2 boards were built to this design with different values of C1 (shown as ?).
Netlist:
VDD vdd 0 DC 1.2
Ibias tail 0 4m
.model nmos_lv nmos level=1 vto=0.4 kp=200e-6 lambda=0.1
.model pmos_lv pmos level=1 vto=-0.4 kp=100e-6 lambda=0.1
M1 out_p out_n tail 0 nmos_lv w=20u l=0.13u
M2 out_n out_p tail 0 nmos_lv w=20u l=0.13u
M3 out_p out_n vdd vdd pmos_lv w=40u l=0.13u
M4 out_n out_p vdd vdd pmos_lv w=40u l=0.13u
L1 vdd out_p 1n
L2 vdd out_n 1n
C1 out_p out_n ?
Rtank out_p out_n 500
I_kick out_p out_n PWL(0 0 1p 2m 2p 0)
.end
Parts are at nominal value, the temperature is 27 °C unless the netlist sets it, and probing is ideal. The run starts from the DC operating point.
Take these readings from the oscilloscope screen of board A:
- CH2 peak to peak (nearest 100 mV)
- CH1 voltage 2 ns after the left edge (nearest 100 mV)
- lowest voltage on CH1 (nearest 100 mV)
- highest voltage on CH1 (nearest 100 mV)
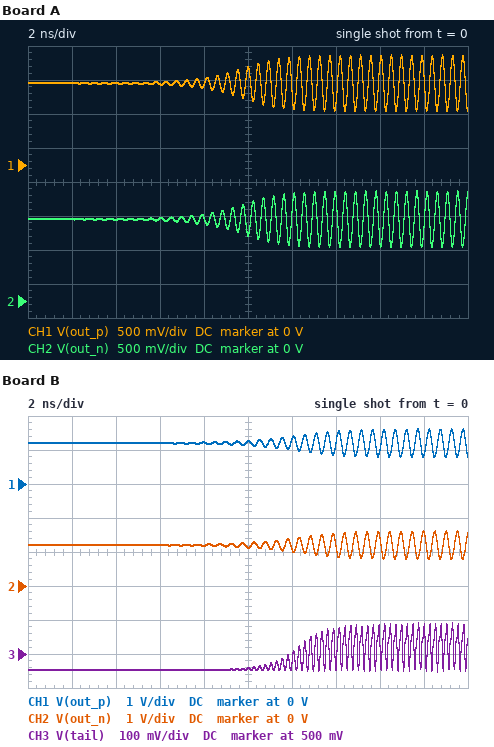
800 mV
1.2 V
800 mV
1.6 V
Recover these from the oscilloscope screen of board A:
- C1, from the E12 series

2.7 pF
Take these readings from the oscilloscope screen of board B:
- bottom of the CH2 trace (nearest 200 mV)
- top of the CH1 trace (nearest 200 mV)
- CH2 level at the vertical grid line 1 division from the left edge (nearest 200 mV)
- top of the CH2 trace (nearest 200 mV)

800 mV
1.6 V
1.2 V
1.6 V
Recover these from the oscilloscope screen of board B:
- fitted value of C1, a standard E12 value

3.3 pF
